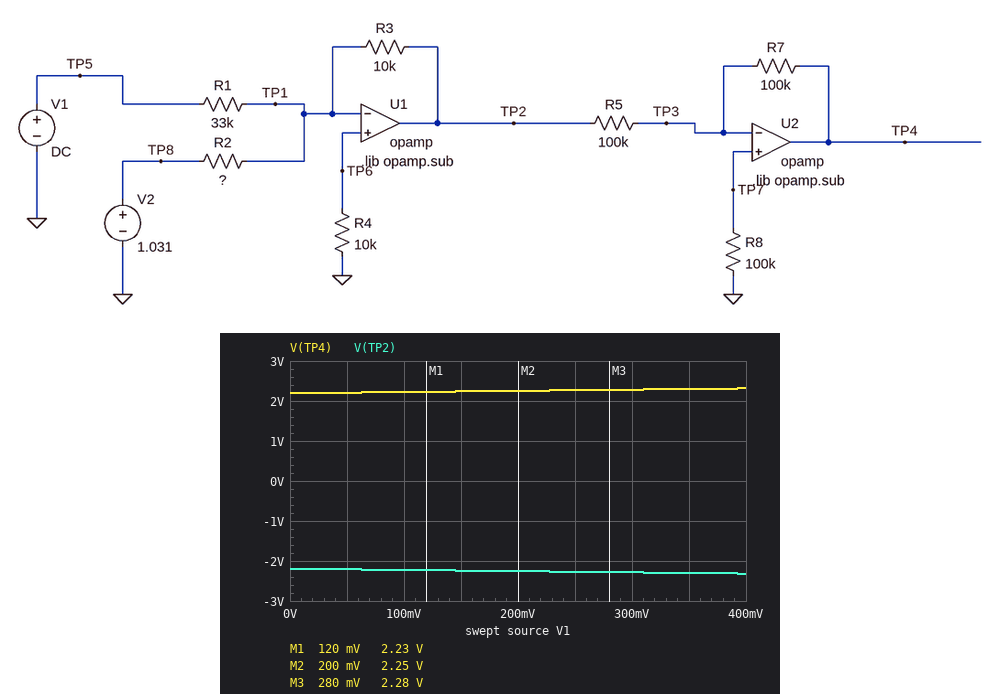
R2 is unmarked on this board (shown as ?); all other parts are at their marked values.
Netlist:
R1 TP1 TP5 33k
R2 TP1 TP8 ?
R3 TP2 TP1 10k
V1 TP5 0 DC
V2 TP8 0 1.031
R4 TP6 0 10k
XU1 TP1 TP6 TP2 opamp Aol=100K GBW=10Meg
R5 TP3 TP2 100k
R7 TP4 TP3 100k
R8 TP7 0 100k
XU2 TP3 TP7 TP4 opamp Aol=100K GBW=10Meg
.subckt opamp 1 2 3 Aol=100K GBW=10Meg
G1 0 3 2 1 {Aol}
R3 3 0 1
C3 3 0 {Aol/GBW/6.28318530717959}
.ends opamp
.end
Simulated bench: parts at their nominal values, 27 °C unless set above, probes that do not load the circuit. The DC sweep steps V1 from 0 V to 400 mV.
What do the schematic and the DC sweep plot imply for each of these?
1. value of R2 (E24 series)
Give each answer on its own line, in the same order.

4.7 kΩ
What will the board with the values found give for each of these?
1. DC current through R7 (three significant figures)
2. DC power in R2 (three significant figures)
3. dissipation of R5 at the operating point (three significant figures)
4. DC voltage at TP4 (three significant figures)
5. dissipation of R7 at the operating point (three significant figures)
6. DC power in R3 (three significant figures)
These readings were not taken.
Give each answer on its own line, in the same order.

21.9 µA
226 µW
48.1 µW
2.19 V
48.1 µW
481 µW
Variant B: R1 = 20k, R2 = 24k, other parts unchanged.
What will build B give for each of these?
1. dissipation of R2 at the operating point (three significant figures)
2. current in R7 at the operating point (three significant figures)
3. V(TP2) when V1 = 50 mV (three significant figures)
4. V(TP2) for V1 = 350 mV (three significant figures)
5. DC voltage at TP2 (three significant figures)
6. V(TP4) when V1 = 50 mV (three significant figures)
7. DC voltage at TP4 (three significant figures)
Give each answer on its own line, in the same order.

44.3 µW
4.30 µA
-455 mV
-605 mV
-430 mV
455 mV
430 mV
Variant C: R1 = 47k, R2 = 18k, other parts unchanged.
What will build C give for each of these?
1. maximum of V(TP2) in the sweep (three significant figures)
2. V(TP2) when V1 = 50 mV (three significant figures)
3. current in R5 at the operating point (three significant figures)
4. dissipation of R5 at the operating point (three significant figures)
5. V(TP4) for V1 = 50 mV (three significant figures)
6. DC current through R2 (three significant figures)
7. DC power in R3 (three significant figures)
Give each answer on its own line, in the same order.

-573 mV
-583 mV
5.73 µA
3.28 µW
583 mV
57.3 µA
32.8 µW
